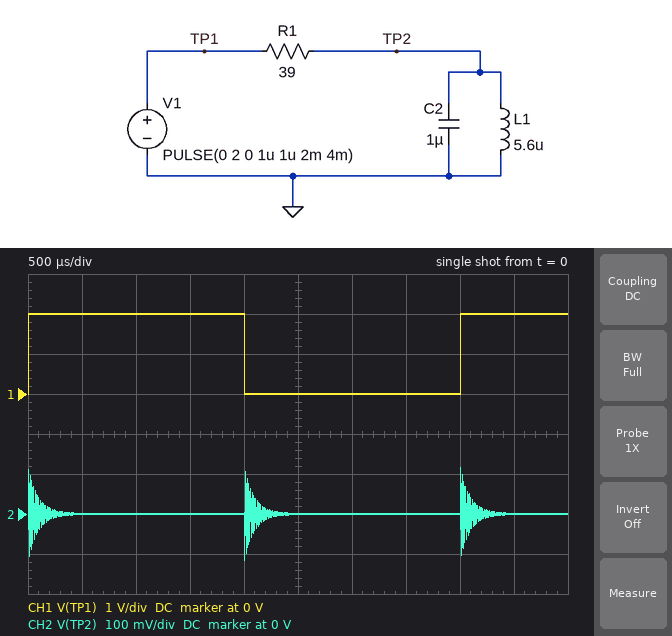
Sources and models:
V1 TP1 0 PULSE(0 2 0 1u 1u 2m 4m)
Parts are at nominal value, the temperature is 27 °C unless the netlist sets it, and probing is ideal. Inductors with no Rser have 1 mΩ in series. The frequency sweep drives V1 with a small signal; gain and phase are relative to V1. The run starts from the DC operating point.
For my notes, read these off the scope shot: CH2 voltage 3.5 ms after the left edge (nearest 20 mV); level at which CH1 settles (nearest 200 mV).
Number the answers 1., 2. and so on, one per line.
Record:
1. 0 V
2. 2.0 V
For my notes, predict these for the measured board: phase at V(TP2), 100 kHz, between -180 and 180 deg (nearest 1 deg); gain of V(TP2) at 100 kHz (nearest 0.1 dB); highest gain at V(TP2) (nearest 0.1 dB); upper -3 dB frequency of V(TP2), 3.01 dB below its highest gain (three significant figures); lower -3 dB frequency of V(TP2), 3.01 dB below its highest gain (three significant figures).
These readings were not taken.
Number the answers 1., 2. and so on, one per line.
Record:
1. -86 deg
2. -22.6 dB
3. -0.1 dB
4. 69.3 kHz
5. 65.2 kHz
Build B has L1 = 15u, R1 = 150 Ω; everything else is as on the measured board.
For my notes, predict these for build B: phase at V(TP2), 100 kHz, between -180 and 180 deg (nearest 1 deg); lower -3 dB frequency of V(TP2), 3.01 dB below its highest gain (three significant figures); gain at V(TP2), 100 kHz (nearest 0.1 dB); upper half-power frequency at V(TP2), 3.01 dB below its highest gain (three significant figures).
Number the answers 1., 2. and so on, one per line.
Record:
1. -89 deg
2. 40.6 kHz
3. -37.9 dB
4. 41.6 kHz
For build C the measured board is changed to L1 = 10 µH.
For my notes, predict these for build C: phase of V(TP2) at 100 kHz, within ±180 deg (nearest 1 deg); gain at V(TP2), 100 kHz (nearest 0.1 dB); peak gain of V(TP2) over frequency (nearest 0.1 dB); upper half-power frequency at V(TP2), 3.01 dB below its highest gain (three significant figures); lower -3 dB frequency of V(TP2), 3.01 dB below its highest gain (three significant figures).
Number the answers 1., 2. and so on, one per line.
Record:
1. -87 deg
2. -25.3 dB
3. 0 dB
4. 52.4 kHz
5. 48.3 kHz
